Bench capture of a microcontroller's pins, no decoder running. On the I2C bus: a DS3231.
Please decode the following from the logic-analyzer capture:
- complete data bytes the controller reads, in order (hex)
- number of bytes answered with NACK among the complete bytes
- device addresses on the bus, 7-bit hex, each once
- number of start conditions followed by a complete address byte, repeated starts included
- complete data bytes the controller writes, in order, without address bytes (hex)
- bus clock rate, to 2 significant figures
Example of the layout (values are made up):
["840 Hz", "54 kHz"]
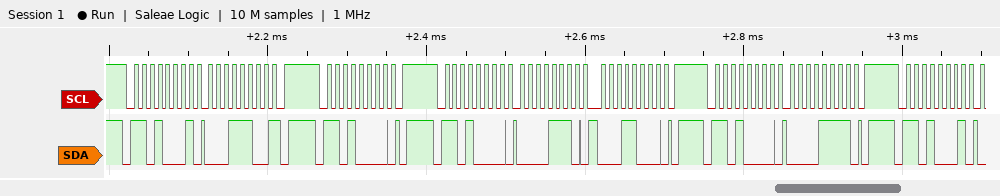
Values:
["1C", "1", "0x68", "5", "0E 18 0F", "100 kHz"]
